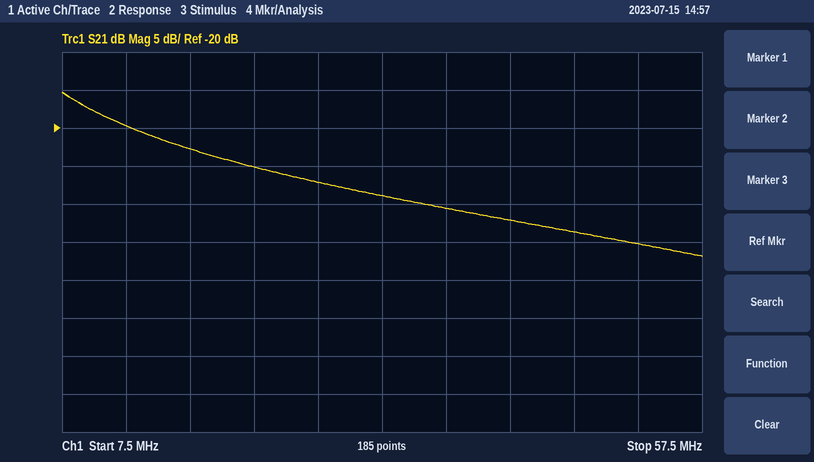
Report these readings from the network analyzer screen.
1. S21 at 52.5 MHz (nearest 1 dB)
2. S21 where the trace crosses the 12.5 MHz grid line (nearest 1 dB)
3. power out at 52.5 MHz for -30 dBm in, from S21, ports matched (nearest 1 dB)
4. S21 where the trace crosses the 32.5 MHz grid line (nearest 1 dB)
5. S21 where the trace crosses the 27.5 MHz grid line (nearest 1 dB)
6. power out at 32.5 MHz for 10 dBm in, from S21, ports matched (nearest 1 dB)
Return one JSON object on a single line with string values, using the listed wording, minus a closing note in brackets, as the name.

{"S21 at 52.5 MHz": "-35 dB", "S21 where the trace crosses the 12.5 MHz grid line": "-20 dB", "power out at 52.5 MHz for -30 dBm in, from S21, ports matched": "-65 dBm", "S21 where the trace crosses the 32.5 MHz grid line": "-29 dB", "S21 where the trace crosses the 27.5 MHz grid line": "-27 dB", "power out at 32.5 MHz for 10 dBm in, from S21, ports matched": "-19 dBm"}
